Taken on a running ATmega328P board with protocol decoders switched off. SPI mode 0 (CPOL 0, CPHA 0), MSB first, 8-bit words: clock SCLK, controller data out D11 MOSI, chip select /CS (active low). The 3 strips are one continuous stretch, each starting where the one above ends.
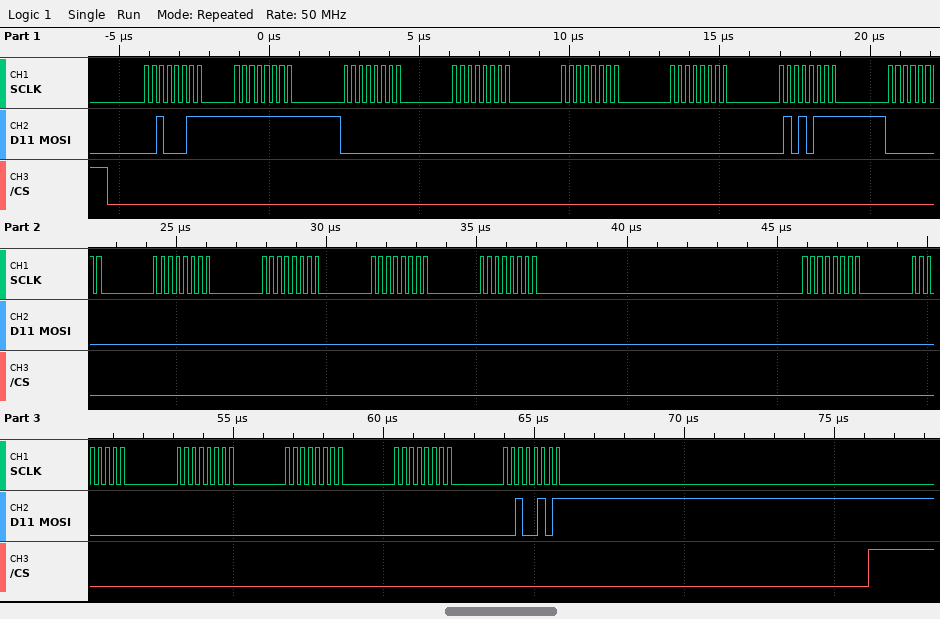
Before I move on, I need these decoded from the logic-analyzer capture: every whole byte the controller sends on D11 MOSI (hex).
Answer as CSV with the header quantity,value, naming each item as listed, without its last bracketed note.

quantity,value
every whole byte the controller sends on D11 MOSI,23 FF 00 00 00 00 57 00 00 00 00 00 00 00 00 00 00 25
